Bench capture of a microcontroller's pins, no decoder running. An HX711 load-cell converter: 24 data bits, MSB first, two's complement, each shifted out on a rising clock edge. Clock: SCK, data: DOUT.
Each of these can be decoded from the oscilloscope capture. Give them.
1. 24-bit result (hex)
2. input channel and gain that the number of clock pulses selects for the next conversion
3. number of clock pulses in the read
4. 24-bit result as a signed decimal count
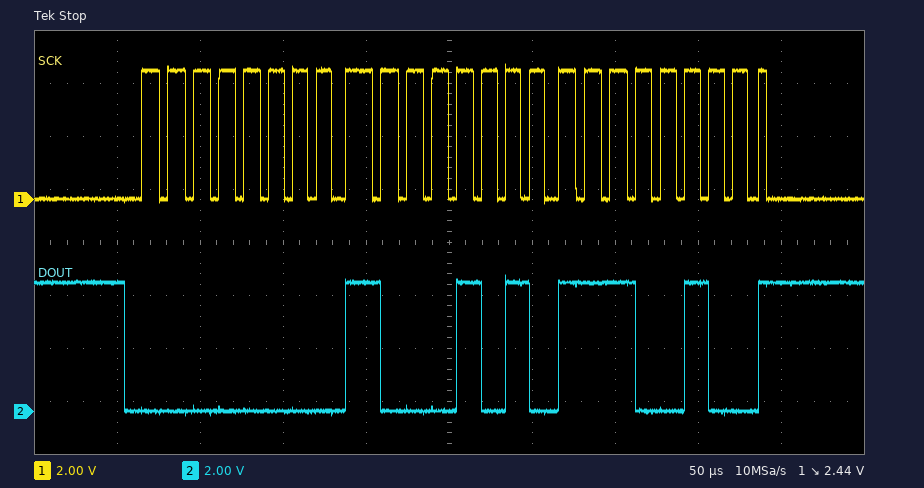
0x008AE4
channel A, gain 128
25
35556
